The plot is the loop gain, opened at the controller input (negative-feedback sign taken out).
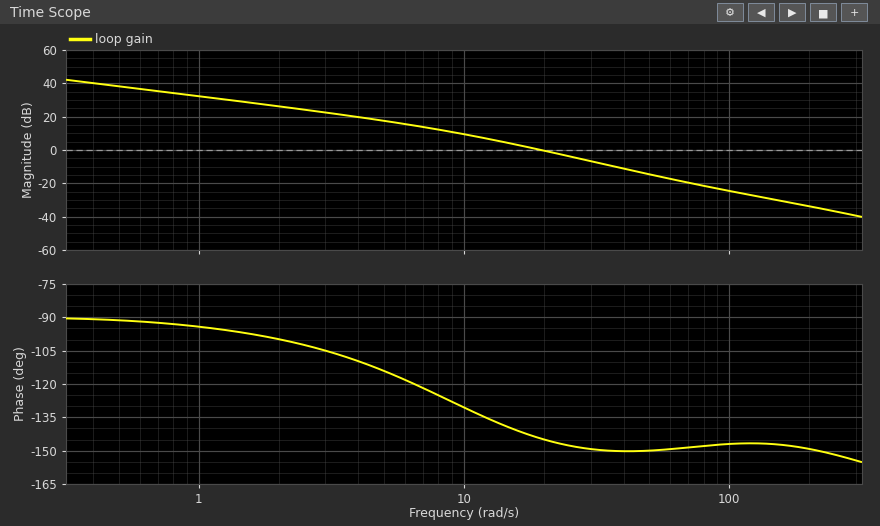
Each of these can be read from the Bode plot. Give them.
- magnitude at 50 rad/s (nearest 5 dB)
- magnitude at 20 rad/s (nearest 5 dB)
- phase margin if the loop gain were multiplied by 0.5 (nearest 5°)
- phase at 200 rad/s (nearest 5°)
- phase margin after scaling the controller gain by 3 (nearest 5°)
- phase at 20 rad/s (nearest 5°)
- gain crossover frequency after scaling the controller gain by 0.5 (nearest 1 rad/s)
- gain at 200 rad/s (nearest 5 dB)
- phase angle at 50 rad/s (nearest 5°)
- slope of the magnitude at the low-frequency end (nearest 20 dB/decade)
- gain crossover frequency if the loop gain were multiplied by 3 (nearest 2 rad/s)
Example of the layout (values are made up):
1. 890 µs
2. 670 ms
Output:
1. -15 dB
2. 0 dB
3. 45°
4. -150°
5. 30°
6. -145°
7. 13 rad/s
8. -35 dB
9. -150°
10. -20 dB/decade
11. 36 rad/s
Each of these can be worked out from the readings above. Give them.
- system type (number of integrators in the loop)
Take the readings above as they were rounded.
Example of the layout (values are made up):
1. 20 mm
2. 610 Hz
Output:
1. 1
